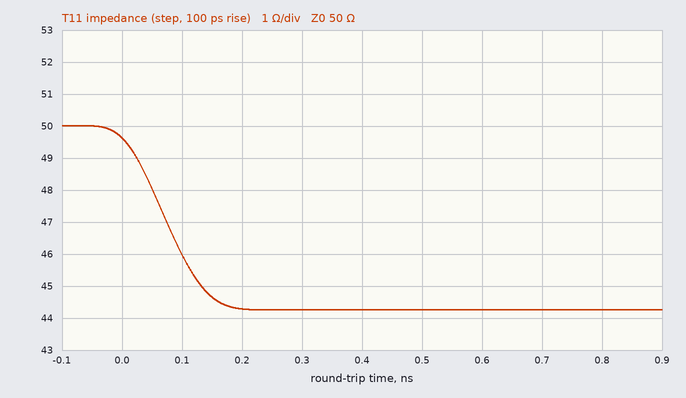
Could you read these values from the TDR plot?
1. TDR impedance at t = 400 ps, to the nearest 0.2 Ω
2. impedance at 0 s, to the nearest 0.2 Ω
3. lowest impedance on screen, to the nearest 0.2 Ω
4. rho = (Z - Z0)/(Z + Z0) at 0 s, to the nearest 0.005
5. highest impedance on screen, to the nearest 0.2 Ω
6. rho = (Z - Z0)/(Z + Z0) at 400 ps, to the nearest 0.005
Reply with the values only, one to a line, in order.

44.2 Ω
49.6 Ω
44.2 Ω
-0.005
50.0 Ω
-0.060
